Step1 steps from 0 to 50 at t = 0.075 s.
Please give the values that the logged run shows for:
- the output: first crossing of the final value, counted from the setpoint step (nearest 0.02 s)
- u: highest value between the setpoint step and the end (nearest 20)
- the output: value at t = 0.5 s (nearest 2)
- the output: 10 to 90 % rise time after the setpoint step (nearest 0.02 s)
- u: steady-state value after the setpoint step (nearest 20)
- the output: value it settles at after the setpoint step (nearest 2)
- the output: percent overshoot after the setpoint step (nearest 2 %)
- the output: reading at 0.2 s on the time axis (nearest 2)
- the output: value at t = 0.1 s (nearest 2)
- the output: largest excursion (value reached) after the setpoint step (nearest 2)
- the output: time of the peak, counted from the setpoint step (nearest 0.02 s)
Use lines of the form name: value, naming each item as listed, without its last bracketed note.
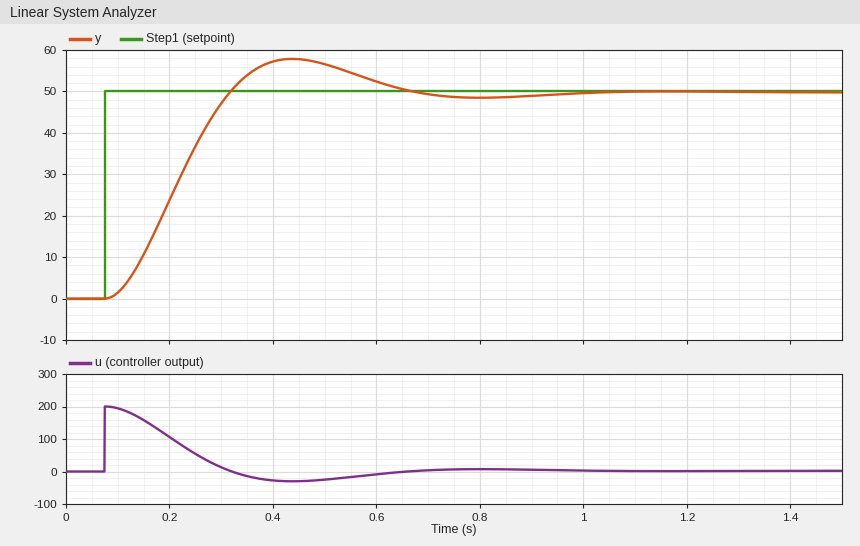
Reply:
the output: first crossing of the final value, counted from the setpoint step: 0.24 s
u: highest value between the setpoint step and the end: 200
the output: value at t = 0.5 s: 56
the output: 10 to 90 % rise time after the setpoint step: 0.16 s
u: steady-state value after the setpoint step: 0
the output: value it settles at after the setpoint step: 50
the output: percent overshoot after the setpoint step: 16 %
the output: reading at 0.2 s on the time axis: 24
the output: value at t = 0.1 s: 2
the output: largest excursion (value reached) after the setpoint step: 58
the output: time of the peak, counted from the setpoint step: 0.36 s
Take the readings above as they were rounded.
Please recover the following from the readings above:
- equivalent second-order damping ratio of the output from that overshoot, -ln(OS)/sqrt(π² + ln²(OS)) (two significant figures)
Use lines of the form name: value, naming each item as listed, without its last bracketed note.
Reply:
equivalent second-order damping ratio of the output from that overshoot, -ln(OS)/sqrt(π² + ln²(OS)): 0.50
